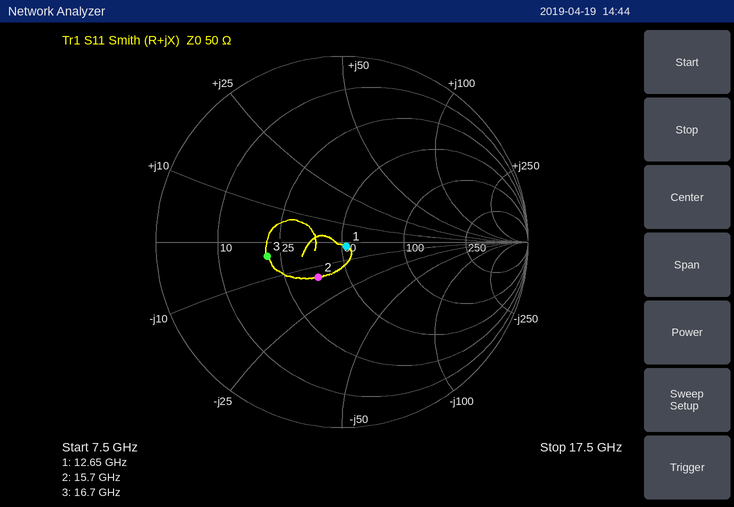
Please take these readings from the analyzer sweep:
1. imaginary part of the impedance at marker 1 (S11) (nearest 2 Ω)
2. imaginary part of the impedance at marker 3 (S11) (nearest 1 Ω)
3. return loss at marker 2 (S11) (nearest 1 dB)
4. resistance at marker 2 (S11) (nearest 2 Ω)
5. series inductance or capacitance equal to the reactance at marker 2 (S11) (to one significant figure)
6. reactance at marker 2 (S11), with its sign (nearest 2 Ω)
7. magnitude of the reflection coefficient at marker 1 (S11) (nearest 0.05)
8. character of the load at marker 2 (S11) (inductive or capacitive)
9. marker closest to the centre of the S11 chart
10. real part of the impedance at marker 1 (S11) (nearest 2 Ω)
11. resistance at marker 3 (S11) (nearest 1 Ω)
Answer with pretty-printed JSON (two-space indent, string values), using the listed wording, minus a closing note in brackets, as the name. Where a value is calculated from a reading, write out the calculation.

{
  "imaginary part of the impedance at marker 1 (S11)": "-2 Ω",
  "imaginary part of the impedance at marker 3 (S11)": "-4 Ω",
  "return loss at marker 2 (S11)": "13 dB",
  "resistance at marker 2 (S11)": "36 Ω",
  "series inductance or capacitance equal to the reactance at marker 2 (S11)": "C = 1/(2π × 15.7 GHz × 14 Ω) ≈ 724 fF, so 700 fF to one significant figure",
  "reactance at marker 2 (S11), with its sign": "-14 Ω",
  "magnitude of the reflection coefficient at marker 1 (S11)": "0.05",
  "character of the load at marker 2 (S11)": "capacitive",
  "marker closest to the centre of the S11 chart": "marker 1",
  "real part of the impedance at marker 1 (S11)": "52 Ω",
  "resistance at marker 3 (S11)": "21 Ω"
}
